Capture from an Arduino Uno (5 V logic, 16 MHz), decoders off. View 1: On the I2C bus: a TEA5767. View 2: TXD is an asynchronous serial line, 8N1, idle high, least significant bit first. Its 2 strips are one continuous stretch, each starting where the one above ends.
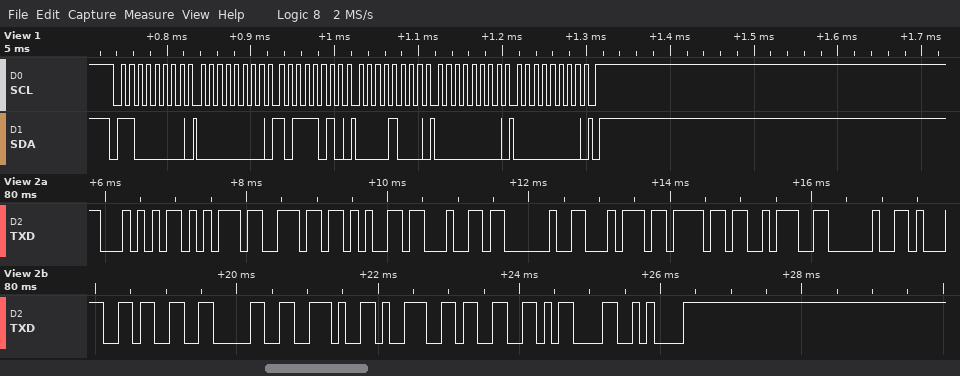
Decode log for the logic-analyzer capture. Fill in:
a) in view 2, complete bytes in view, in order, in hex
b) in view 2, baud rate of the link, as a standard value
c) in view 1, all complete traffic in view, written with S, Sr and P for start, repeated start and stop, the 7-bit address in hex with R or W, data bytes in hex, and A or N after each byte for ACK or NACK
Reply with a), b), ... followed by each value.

a) 0x54 0x75 0x6E 0x65 0x64 0x20 0x74 0x6F 0x3A 0x20 0x31 0x33 0x30 0x2E 0x39 0x33 0x0D 0x0A
b) 9600 baud
c) S 60W A 00 A BA A 08 A 00 A 00 A P
